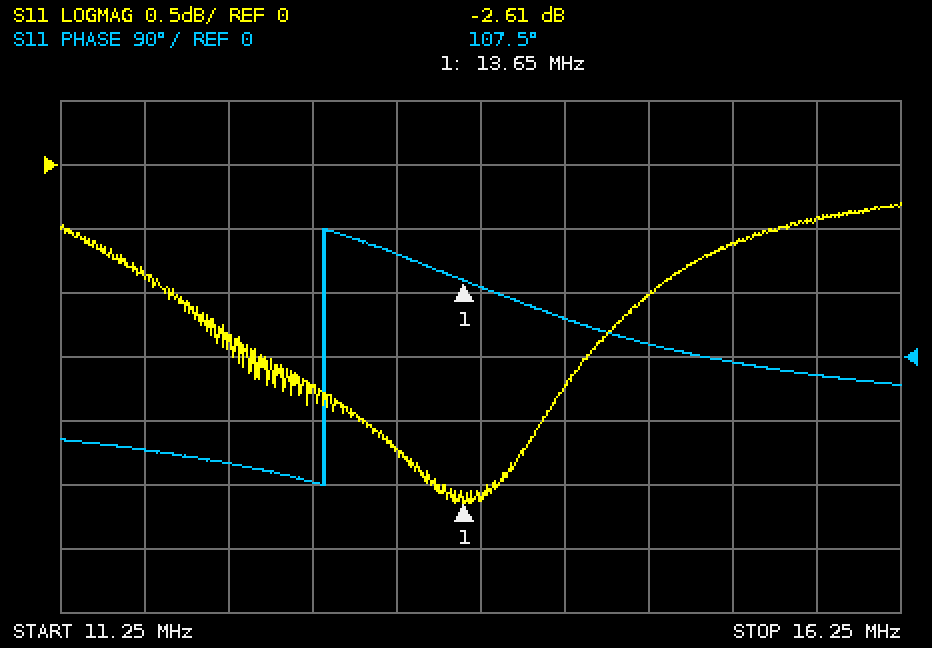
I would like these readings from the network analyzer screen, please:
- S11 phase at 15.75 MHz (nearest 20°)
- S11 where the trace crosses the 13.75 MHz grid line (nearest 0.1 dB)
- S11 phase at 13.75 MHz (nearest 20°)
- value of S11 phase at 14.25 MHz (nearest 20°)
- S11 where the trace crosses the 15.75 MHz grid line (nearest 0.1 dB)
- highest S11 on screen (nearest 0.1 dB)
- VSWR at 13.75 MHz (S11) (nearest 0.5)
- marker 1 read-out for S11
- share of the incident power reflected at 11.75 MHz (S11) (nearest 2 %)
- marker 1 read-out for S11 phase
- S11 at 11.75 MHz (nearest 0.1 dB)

-20°
-2.6 dB
100°
60°
-0.4 dB
-0.3 dB
6.5
-2.61 dB
82 %
107.5°
-0.9 dB
